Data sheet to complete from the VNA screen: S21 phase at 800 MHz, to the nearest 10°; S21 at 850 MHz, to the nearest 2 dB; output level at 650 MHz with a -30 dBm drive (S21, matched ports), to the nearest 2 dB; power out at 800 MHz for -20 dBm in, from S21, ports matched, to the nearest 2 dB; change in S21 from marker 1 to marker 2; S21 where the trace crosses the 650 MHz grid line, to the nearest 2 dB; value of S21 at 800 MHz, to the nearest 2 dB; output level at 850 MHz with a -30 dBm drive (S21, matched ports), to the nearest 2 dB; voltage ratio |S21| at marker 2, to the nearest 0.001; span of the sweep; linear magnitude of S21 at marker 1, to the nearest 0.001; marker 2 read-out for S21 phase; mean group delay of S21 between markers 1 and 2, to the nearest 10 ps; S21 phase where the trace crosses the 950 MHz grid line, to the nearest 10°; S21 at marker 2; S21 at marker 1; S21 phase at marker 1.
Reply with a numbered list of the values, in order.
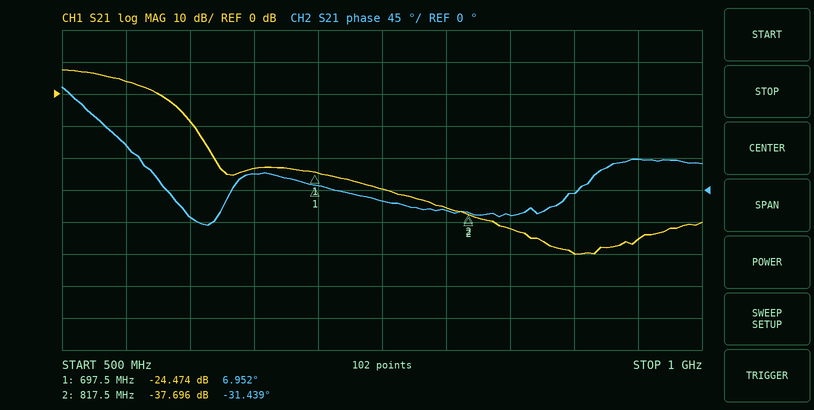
1. -30°
2. -42 dB
3. -54 dBm
4. -56 dBm
5. -13.222 dB
6. -24 dB
7. -36 dB
8. -72 dBm
9. 0.013
10. 500 MHz
11. 0.060
12. -31.439°
13. 890 ps
14. 40°
15. -37.696 dB
16. -24.474 dB
17. 6.952°
